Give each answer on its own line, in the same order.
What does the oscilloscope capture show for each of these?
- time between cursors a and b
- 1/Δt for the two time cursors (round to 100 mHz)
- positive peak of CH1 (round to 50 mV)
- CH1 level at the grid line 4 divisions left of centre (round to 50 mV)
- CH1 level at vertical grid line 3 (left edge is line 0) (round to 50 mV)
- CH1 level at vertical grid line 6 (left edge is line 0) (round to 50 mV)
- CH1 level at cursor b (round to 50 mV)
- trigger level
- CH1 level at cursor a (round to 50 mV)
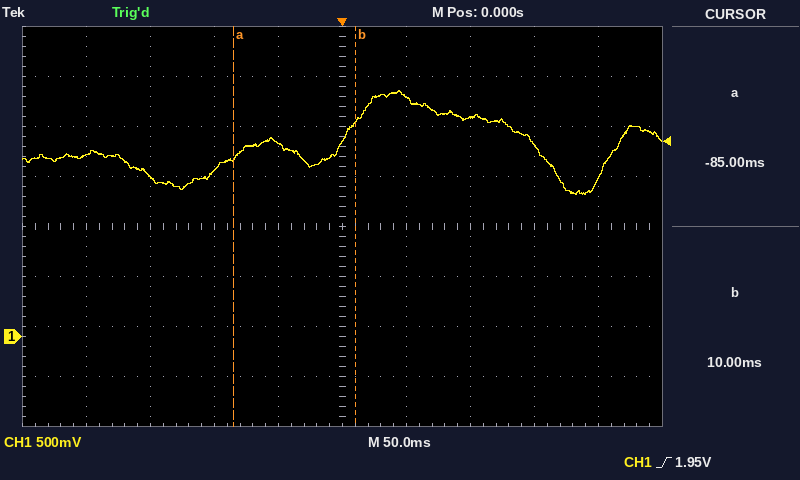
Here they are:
95 ms
10.5 Hz
2.45 V
1.80 V
1.65 V
2.40 V
2.15 V
1.95 V
1.80 V
